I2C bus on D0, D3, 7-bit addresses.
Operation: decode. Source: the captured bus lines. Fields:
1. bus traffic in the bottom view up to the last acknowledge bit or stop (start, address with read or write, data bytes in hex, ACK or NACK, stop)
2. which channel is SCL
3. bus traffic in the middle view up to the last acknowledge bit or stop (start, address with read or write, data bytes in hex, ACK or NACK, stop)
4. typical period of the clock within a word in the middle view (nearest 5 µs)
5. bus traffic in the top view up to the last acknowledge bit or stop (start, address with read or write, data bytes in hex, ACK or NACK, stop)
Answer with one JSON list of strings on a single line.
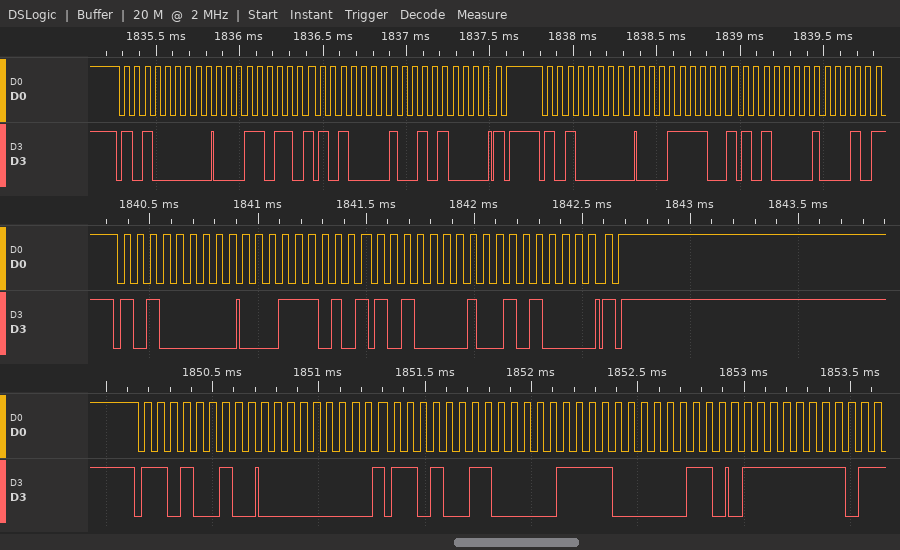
["start, address 69 write ACK, 00 ACK, repeated start, address 69 read ACK, 0F ACK, 06 ACK, FF ACK", "D0", "start, address 50 write ACK, 1D ACK, repeated start, address 50 read ACK, 50 NACK, stop", "60 µs", "start, address 50 write ACK, 1B ACK, repeated start, address 50 read ACK, 50 NACK, stop, start, address 50 write ACK, 1E ACK, repeated start, address 50 read ACK"]
